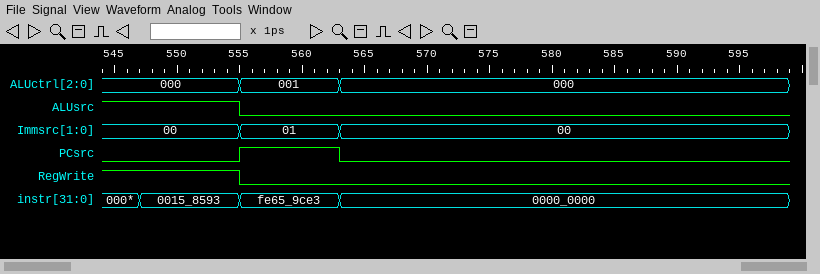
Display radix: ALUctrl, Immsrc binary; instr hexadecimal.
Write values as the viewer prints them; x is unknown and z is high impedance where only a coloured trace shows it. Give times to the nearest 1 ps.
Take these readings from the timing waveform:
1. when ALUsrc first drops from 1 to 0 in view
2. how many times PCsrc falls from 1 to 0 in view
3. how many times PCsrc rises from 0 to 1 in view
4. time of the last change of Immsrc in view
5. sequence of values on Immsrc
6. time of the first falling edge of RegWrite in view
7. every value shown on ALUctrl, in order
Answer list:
555 ps
1
1
563 ps
00, 01, 00
555 ps
000, 001, 000
